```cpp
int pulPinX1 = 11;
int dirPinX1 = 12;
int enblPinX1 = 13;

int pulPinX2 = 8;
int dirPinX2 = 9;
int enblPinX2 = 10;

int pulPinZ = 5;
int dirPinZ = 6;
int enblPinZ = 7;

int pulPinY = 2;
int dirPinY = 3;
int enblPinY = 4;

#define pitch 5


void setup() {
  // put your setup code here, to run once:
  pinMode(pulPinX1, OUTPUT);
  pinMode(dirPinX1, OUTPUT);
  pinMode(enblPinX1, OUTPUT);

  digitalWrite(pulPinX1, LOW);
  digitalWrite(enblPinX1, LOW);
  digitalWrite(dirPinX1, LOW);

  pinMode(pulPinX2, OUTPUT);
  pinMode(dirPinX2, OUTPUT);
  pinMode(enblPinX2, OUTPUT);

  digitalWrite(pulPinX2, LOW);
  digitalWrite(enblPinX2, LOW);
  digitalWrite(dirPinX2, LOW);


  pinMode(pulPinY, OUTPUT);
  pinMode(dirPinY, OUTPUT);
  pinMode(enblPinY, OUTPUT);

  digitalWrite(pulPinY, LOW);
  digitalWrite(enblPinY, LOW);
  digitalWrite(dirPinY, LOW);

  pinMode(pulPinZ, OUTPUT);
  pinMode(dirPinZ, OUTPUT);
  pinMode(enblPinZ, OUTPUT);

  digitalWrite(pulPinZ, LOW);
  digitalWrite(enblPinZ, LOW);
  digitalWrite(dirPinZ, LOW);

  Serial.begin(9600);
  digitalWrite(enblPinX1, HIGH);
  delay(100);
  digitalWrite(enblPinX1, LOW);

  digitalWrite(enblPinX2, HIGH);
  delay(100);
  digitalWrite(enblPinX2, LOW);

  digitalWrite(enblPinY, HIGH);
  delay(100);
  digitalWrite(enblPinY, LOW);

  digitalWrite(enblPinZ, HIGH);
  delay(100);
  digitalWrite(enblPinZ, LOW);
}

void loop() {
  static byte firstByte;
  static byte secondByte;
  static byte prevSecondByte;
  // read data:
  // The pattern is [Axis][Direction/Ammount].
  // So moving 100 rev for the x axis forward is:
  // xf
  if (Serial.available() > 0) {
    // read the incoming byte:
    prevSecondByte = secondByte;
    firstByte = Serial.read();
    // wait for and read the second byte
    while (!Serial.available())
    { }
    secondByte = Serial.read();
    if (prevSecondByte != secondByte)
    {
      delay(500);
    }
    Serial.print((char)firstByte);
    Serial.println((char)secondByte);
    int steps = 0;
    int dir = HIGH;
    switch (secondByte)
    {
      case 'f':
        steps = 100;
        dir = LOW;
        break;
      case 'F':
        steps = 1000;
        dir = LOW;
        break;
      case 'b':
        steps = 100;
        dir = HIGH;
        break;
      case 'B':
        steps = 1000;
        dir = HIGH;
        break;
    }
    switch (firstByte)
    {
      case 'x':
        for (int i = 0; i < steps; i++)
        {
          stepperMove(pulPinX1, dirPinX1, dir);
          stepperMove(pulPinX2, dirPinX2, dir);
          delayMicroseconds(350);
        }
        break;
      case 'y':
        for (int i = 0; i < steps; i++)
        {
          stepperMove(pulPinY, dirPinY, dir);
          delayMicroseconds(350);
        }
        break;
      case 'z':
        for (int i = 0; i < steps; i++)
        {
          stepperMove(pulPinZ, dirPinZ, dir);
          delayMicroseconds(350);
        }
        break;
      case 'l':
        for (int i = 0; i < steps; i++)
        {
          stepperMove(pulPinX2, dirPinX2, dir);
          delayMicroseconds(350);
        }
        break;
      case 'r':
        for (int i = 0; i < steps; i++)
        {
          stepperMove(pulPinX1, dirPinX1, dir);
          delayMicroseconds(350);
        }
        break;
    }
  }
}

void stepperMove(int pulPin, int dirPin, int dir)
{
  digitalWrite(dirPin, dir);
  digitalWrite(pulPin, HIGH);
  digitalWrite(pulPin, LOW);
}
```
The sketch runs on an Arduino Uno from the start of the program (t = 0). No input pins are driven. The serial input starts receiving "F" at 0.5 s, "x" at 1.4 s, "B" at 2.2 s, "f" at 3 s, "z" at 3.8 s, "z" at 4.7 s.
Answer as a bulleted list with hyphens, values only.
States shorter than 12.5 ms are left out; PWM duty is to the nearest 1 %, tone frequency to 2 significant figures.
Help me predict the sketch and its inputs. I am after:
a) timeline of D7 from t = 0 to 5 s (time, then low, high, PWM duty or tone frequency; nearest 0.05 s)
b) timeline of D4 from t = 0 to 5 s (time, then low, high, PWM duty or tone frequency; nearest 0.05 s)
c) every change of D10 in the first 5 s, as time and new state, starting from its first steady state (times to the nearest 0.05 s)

- 0 s low; 0.3 s high; 0.4 s low
- 0 s low; 0.2 s high; 0.3 s low
- 0 s low; 0.1 s high; 0.2 s low
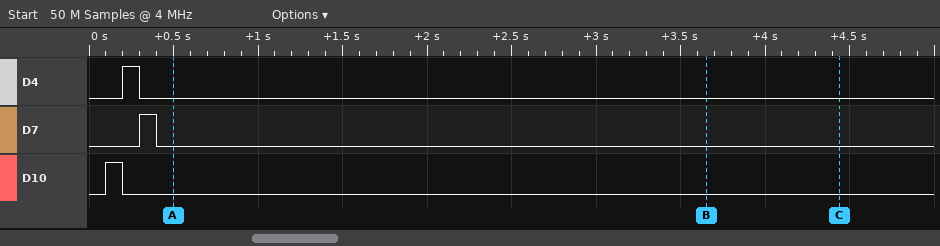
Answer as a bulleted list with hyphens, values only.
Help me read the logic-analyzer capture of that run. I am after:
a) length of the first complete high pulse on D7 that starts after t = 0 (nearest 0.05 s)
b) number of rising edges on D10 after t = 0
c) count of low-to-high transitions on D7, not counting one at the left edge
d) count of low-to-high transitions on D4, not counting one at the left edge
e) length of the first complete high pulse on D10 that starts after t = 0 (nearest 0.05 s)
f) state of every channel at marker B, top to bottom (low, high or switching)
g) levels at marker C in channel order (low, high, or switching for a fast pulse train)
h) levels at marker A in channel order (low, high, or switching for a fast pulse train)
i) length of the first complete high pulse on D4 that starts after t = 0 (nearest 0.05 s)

- 0.10 s
- 1
- 1
- 1
- 0.10 s
- D4 low, D7 low, D10 low
- D4 low, D7 low, D10 low
- D4 low, D7 low, D10 low
- 0.10 s
